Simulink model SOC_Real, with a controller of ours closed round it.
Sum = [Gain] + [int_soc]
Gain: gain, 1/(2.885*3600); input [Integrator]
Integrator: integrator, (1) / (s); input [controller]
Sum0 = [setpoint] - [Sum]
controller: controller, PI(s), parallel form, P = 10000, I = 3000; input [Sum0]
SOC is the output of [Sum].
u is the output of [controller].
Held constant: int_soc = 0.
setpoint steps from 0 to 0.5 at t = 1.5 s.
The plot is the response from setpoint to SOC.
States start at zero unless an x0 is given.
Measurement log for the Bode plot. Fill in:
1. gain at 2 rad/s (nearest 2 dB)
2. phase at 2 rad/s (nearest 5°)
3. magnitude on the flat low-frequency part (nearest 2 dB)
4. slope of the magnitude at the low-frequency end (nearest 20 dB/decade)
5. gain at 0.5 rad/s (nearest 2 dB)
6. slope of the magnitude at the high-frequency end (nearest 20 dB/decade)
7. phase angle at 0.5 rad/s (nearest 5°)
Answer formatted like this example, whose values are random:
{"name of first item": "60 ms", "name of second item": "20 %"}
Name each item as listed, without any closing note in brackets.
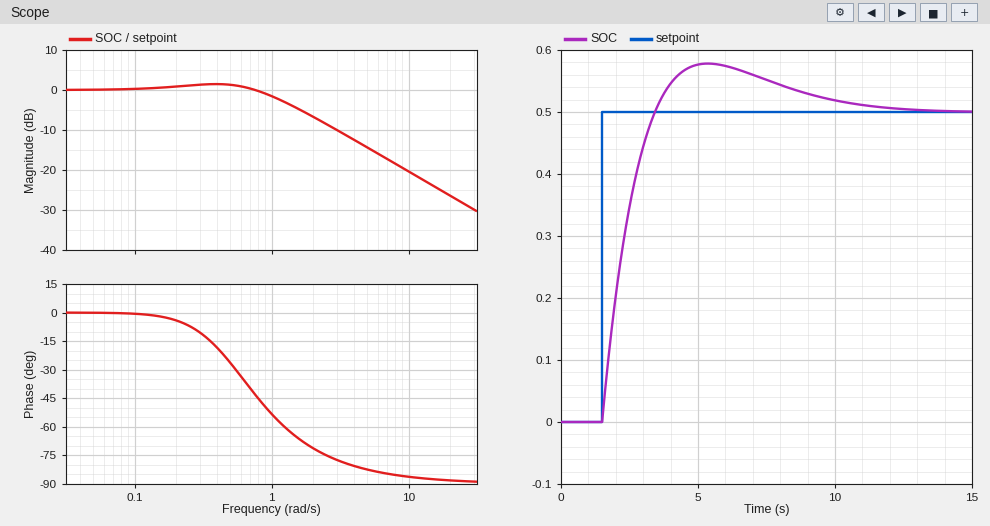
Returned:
{"gain at 2 rad/s": "-6 dB", "phase at 2 rad/s": "-70°", "magnitude on the flat low-frequency part": "0 dB", "slope of the magnitude at the low-frequency end": "0 dB/decade", "gain at 0.5 rad/s": "2 dB", "slope of the magnitude at the high-frequency end": "-20 dB/decade", "phase angle at 0.5 rad/s": "-25°"}
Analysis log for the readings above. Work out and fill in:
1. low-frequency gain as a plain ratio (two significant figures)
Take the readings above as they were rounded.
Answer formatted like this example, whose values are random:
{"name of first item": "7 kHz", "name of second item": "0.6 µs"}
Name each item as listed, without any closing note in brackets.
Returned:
{"low-frequency gain as a plain ratio": "1.0"}
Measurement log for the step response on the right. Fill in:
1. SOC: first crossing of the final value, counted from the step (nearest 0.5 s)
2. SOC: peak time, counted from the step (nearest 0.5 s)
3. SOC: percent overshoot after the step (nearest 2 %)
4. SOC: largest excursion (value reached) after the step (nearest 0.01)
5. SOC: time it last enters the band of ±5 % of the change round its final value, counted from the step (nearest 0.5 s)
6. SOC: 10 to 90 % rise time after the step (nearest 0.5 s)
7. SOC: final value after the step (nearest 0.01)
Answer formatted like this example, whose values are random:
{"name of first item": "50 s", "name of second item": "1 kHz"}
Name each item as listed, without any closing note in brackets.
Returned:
{"SOC: first crossing of the final value, counted from the step": "2.0 s", "SOC: peak time, counted from the step": "4.0 s", "SOC: percent overshoot after the step": "16 %", "SOC: largest excursion (value reached) after the step": "0.58", "SOC: time it last enters the band of ±5 % of the change round its final value, counted from the step": "8.0 s", "SOC: 10 to 90 % rise time after the step": "1.5 s", "SOC: final value after the step": "0.50"}
